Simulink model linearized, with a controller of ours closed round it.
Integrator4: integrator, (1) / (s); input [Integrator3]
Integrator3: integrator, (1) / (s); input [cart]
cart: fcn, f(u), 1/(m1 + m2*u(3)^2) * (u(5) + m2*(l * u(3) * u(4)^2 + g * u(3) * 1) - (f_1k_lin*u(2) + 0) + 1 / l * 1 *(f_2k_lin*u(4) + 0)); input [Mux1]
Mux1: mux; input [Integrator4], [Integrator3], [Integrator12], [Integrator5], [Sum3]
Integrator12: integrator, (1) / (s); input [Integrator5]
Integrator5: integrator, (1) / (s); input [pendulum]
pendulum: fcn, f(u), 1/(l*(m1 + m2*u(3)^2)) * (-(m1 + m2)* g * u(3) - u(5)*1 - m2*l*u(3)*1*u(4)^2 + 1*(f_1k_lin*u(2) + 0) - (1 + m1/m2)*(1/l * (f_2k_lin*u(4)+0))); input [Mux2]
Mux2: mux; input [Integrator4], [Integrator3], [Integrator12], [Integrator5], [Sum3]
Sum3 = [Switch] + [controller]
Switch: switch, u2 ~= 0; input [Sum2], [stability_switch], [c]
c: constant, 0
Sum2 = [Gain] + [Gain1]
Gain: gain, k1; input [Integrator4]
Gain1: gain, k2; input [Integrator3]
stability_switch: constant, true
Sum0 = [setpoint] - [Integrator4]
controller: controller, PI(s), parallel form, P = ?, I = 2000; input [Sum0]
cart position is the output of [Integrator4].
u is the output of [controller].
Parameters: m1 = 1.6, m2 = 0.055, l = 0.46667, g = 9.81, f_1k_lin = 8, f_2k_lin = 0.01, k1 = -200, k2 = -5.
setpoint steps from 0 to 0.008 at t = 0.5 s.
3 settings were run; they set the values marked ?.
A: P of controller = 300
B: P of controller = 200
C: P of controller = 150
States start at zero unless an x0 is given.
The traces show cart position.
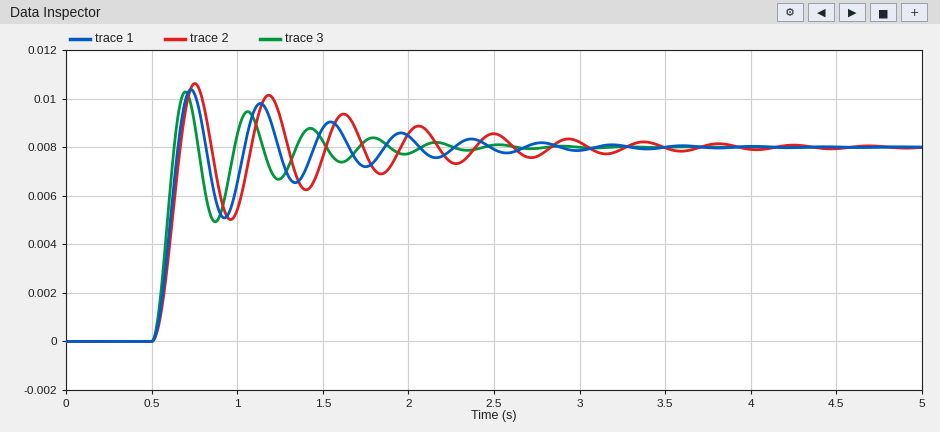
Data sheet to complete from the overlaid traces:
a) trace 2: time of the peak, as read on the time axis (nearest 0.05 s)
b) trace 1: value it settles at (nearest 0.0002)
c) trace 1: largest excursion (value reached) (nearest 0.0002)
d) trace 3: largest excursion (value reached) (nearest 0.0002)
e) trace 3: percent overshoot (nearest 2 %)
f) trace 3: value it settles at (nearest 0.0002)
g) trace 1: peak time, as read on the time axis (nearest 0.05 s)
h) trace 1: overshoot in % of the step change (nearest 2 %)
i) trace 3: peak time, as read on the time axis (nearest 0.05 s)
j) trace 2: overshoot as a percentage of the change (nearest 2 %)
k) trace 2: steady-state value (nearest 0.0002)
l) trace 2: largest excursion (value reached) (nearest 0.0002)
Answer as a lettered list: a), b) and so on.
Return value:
a) 0.75 s
b) 0.0080
c) 0.0104
d) 0.0102
e) 28 %
f) 0.0080
g) 0.75 s
h) 30 %
i) 0.70 s
j) 32 %
k) 0.0080
l) 0.0106
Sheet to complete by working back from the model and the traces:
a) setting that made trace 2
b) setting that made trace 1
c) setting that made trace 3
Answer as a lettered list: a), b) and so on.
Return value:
a) C
b) B
c) A
